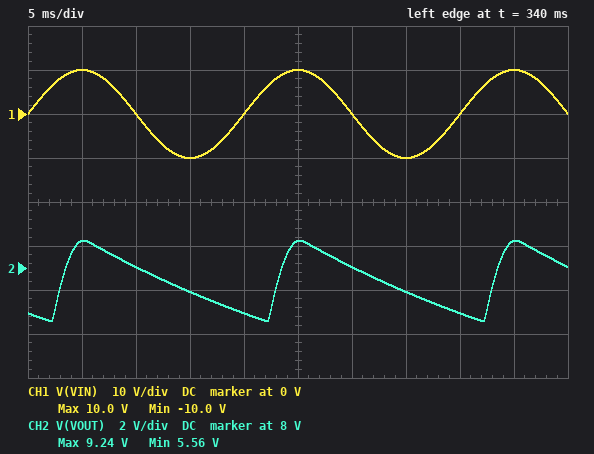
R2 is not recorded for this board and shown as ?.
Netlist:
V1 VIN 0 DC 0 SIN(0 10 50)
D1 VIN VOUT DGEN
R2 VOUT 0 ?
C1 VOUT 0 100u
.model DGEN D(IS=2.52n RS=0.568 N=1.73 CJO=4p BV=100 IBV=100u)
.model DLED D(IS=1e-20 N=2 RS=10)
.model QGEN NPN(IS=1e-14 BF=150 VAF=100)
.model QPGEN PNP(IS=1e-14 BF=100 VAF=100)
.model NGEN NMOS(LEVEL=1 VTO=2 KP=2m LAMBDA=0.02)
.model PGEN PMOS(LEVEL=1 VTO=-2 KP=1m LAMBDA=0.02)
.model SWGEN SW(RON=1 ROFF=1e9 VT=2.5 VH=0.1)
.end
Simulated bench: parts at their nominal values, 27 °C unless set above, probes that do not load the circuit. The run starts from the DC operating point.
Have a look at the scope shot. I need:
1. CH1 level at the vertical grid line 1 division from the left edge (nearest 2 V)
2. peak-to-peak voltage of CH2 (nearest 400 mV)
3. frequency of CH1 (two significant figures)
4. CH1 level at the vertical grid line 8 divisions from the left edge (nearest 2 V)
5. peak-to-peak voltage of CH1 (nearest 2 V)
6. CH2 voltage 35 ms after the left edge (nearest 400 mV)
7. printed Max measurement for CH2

10 V
3.6 V
50 Hz
0 V
20 V
6.8 V
9.24 V
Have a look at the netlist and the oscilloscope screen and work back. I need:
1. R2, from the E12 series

330 Ω
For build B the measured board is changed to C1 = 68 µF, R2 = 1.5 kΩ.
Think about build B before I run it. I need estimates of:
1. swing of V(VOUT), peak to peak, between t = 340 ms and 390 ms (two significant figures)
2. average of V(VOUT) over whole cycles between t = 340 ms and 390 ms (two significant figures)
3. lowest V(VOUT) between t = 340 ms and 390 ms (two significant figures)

1.5 V
8.6 V
7.8 V
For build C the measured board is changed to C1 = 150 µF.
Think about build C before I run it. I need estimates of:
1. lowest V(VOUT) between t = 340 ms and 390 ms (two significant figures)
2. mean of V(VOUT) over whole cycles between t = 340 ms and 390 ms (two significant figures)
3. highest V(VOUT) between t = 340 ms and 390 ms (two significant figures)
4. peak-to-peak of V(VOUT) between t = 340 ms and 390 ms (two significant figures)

6.5 V
7.9 V
9.2 V
2.7 V
